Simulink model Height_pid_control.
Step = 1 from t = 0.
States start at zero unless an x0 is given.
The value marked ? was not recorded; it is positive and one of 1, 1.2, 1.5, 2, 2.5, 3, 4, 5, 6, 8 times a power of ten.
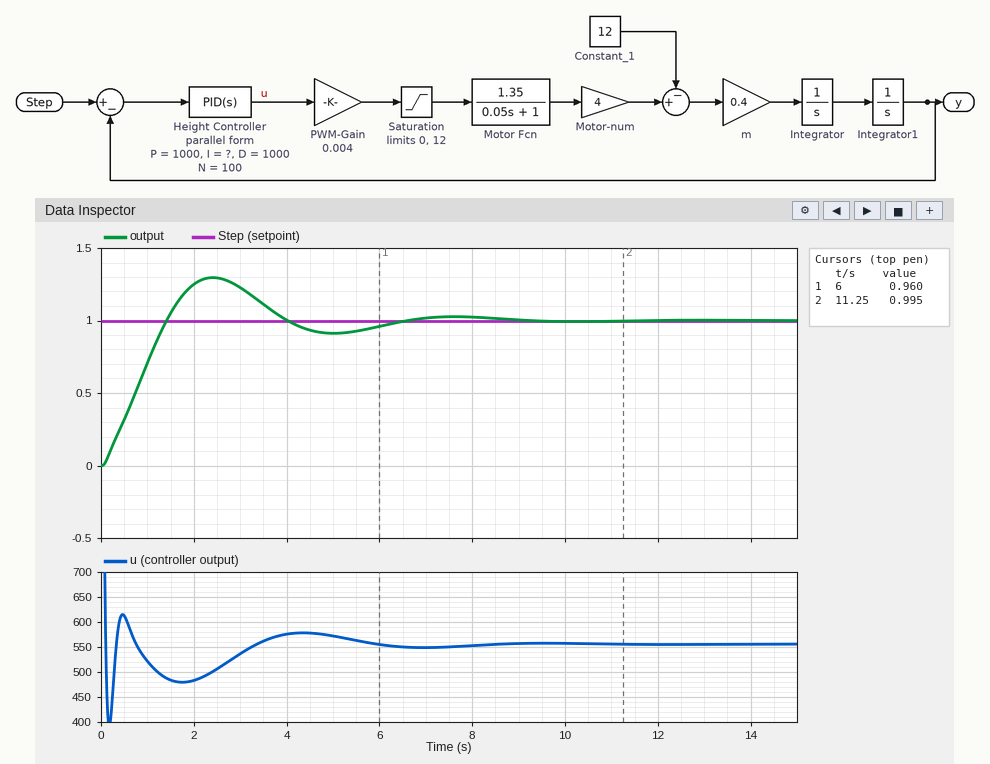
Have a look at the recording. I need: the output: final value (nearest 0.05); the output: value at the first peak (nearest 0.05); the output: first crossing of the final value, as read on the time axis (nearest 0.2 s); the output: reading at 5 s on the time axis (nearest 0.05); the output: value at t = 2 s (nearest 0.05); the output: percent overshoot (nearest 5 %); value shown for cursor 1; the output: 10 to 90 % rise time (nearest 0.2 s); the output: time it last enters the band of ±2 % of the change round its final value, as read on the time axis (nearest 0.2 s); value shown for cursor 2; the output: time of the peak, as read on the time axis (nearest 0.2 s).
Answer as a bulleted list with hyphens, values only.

- 1.00
- 1.30
- 1.4 s
- 0.90
- 1.25
- 30 %
- 0.960
- 1.0 s
- 8.2 s
- 0.995
- 2.4 s
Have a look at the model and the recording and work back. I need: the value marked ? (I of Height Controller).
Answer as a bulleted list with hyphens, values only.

- 1500
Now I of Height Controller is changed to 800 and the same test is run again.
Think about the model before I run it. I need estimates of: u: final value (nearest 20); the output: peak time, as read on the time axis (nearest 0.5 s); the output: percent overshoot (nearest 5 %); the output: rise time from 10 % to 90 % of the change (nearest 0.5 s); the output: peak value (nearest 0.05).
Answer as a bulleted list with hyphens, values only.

- 560
- 3.5 s
- 15 %
- 1.5 s
- 1.15
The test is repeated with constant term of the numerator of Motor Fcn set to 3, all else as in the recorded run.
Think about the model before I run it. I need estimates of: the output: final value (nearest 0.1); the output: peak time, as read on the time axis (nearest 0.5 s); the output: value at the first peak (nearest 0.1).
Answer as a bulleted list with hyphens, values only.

- 1.0
- 2.0 s
- 1.2
